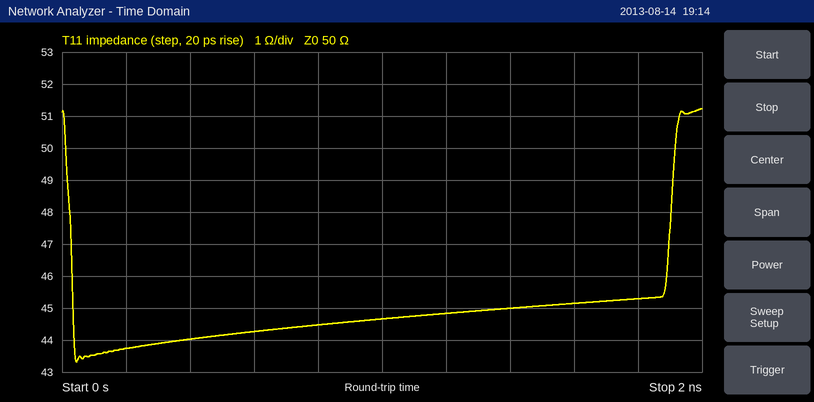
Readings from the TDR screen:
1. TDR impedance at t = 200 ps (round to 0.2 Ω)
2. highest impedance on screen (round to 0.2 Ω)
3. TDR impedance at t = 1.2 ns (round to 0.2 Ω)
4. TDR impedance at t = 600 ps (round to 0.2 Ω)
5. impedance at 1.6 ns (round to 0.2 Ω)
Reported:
43.8 Ω
51.2 Ω
44.8 Ω
44.2 Ω
45.2 Ω
